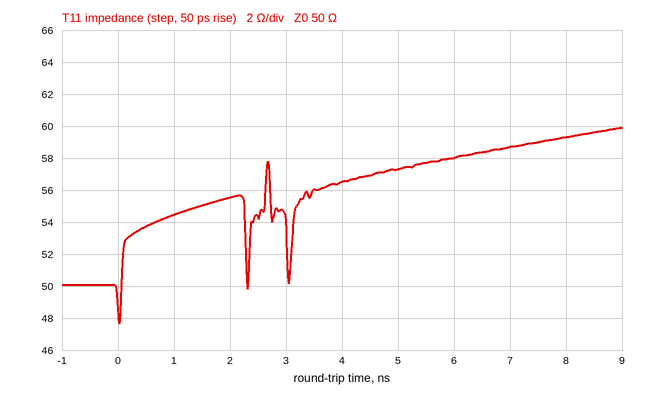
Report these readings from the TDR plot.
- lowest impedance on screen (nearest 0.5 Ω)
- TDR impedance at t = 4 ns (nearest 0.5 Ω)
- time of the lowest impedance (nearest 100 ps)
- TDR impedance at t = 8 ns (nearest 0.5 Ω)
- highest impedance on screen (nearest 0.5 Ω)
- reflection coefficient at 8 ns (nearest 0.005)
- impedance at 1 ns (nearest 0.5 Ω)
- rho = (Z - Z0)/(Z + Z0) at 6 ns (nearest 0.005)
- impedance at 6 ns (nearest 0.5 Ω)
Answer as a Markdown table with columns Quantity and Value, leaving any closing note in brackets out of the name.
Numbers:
| Quantity | Value |
|---|---|
| lowest impedance on screen | 47.5 Ω |
| TDR impedance at t = 4 ns | 56.5 Ω |
| time of the lowest impedance | 0.0 ns |
| TDR impedance at t = 8 ns | 59.5 Ω |
| highest impedance on screen | 60.0 Ω |
| reflection coefficient at 8 ns | +0.085 |
| impedance at 1 ns | 54.5 Ω |
| rho = (Z - Z0)/(Z + Z0) at 6 ns | +0.075 |
| impedance at 6 ns | 58.0 Ω |
